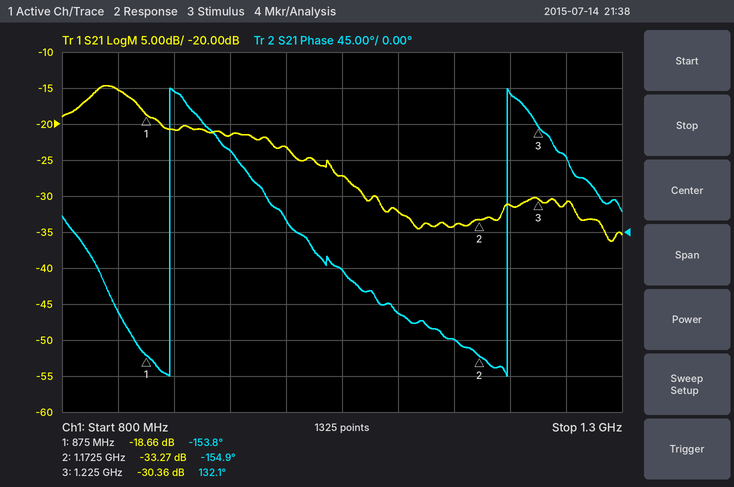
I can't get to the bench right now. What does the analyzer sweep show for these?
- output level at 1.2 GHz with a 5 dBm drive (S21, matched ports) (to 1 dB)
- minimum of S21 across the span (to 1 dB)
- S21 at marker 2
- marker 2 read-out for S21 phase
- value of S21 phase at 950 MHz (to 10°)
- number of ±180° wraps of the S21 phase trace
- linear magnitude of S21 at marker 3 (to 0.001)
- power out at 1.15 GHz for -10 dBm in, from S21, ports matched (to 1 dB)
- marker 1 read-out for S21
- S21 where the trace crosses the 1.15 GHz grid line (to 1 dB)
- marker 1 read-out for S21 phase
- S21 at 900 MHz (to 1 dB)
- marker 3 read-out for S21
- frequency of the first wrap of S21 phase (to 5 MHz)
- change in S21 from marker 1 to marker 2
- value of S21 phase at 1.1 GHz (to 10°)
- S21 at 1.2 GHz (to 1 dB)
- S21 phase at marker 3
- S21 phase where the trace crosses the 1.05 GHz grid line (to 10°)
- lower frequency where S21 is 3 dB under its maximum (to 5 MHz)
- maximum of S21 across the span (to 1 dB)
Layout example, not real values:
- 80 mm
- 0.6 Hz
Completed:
- -26 dBm
- -36 dB
- -33.27 dB
- -154.9°
- 100°
- 2
- 0.030
- -44 dBm
- -18.66 dB
- -34 dB
- -153.8°
- -21 dB
- -30.36 dB
- 895 MHz
- -14.61 dB
- -100°
- -31 dB
- 132.1°
- -50°
- 815 MHz
- -15 dB
